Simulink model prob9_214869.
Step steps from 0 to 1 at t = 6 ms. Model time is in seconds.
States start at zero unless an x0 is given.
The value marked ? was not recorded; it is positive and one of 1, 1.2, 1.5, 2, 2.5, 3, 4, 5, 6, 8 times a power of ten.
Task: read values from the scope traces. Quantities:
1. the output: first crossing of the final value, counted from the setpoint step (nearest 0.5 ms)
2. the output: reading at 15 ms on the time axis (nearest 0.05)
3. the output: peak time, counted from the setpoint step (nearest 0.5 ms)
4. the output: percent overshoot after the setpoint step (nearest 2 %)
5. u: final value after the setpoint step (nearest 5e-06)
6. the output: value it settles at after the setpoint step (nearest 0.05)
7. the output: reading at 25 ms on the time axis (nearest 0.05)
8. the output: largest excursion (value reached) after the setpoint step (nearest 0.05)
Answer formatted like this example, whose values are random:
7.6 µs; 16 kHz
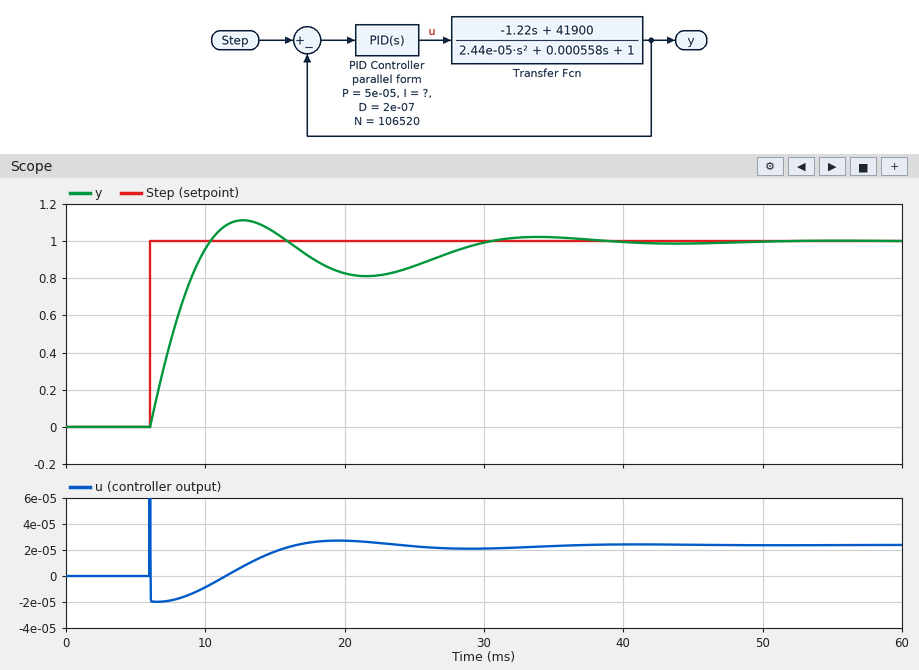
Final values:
4.5 ms; 1.05; 6.5 ms; 12 %; 0.000025; 1.00; 0.85; 1.10
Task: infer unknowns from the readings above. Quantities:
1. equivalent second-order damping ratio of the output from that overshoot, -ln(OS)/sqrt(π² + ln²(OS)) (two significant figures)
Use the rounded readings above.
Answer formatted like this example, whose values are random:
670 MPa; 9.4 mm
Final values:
0.56
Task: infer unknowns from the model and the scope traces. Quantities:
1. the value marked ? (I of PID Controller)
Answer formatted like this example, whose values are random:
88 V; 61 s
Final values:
0.008
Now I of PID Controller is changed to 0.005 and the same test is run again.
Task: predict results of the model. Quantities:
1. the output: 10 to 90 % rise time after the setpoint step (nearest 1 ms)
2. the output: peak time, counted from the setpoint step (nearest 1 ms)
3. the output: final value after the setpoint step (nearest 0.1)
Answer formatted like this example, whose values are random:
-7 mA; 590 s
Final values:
3 ms; 6 ms; 1.0
